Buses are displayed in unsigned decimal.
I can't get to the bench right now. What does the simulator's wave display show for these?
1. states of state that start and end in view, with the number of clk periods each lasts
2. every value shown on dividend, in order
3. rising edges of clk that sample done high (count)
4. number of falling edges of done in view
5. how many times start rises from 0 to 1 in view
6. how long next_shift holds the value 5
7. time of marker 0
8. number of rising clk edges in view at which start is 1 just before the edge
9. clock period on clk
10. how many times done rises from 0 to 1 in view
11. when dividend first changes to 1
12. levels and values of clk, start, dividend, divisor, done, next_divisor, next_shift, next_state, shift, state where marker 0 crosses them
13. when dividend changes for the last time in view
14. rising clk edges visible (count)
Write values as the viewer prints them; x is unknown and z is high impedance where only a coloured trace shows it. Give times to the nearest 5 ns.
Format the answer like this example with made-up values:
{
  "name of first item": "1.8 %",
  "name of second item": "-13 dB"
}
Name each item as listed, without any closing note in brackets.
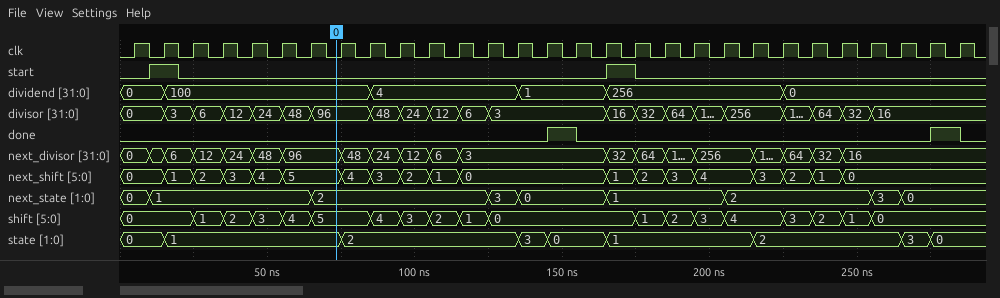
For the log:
{
  "states of state that start and end in view, with the number of clk periods each lasts": "1: 6, 2: 6, 3: 1, 0: 2, 1: 5, 2: 5, 3: 1",
  "every value shown on dividend, in order": "0, 100, 4, 1, 256, 0",
  "rising edges of clk that sample done high": "2",
  "number of falling edges of done in view": "2",
  "how many times start rises from 0 to 1 in view": "2",
  "how long next_shift holds the value 5": "20 ns",
  "time of marker 0": "75 ns",
  "number of rising clk edges in view at which start is 1 just before the edge": "2",
  "clock period on clk": "10 ns",
  "how many times done rises from 0 to 1 in view": "2",
  "when dividend first changes to 1": "135 ns",
  "levels and values of clk, start, dividend, divisor, done, next_divisor, next_shift, next_state, shift, state where marker 0 crosses them": "clk=0, start=0, dividend=100, divisor=96, done=0, next_divisor=96, next_shift=5, next_state=2, shift=5, state=1",
  "when dividend changes for the last time in view": "225 ns",
  "rising clk edges visible": "29"
}
